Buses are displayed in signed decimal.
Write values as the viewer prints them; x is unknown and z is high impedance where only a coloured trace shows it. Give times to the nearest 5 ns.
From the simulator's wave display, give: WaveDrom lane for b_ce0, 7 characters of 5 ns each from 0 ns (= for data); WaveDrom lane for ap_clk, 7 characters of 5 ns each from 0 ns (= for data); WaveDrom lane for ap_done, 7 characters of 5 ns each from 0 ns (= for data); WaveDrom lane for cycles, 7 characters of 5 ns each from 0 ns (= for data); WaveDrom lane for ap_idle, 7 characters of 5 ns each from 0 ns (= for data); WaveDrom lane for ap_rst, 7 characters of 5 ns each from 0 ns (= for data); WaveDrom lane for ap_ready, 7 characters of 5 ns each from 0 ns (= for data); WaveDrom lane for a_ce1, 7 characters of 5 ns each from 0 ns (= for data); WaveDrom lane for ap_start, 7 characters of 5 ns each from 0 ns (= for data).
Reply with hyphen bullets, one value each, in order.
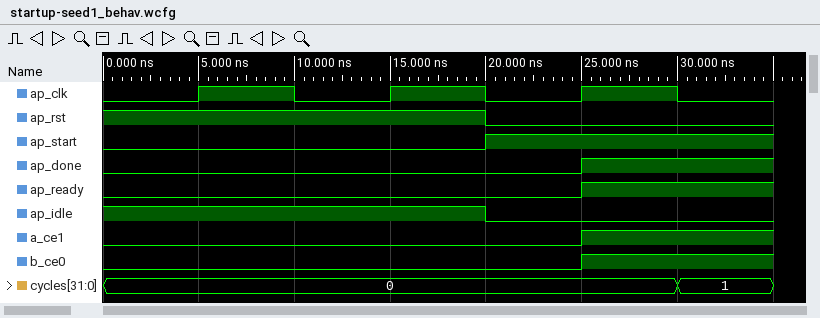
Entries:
- {name: 'b_ce0', wave: '0....1.'}
- {name: 'ap_clk', wave: '0101010'}
- {name: 'ap_done', wave: '0....1.'}
- {name: 'cycles', wave: '=.....=', data: '0 1'}
- {name: 'ap_idle', wave: '1...0..'}
- {name: 'ap_rst', wave: '1...0..'}
- {name: 'ap_ready', wave: '0....1.'}
- {name: 'a_ce1', wave: '0....1.'}
- {name: 'ap_start', wave: '0...1..'}
